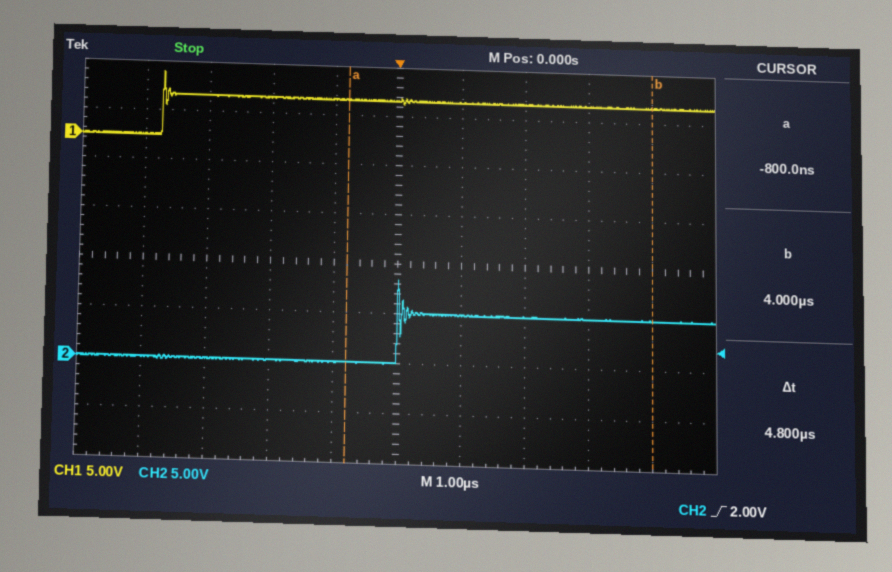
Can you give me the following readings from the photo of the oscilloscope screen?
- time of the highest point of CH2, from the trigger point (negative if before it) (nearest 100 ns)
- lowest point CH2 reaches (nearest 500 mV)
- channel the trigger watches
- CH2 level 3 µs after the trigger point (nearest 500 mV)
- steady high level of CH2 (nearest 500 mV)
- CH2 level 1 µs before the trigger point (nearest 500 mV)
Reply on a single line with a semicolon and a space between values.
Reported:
0.0 µs; 0.0 V; CH2; 5.0 V; 5.0 V; 0.0 V
